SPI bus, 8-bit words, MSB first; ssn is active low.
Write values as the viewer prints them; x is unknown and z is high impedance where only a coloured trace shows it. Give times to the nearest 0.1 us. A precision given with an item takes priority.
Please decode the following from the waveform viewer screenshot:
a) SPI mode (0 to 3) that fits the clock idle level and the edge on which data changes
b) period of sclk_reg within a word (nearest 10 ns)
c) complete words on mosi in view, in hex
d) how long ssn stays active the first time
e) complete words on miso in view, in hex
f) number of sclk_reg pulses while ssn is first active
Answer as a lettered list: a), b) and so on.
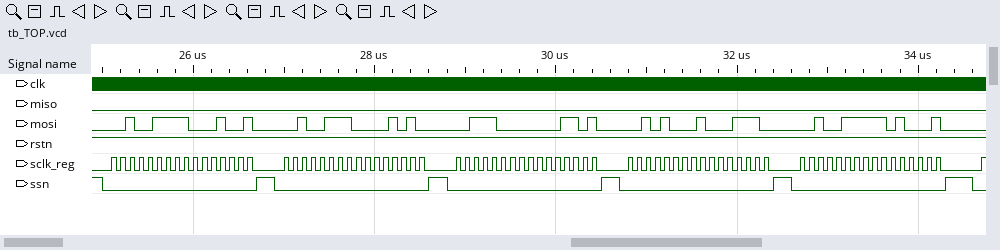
a) 0
b) 100 ns
c) 27, 89, 27, 0A, 38, 0D, 28, 8E, 27, D1
d) 1.7 us
e) 00, 00, 00, 00, 00, 00, 00, 00, 00, 00
f) 16
